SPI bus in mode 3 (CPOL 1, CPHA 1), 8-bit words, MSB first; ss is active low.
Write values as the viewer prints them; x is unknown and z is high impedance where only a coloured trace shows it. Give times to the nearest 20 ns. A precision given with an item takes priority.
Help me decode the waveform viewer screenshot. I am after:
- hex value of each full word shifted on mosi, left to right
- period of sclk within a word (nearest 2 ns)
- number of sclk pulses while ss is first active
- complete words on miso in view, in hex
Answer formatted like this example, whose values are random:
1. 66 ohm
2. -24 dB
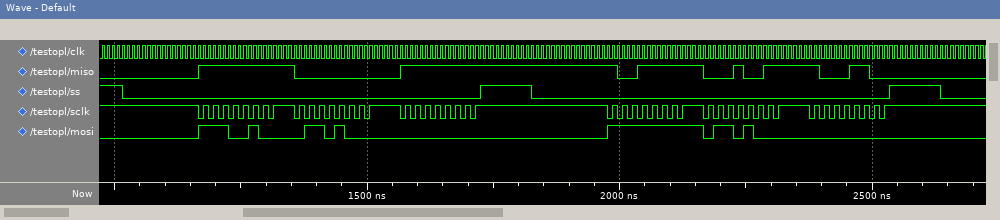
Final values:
1. E4, 68, 00, FF, 68, 00
2. 20 ns
3. 24
4. FF, 00, FF, 9F, 13, 8C
